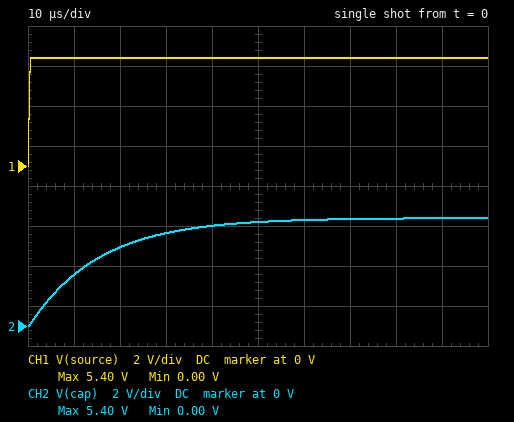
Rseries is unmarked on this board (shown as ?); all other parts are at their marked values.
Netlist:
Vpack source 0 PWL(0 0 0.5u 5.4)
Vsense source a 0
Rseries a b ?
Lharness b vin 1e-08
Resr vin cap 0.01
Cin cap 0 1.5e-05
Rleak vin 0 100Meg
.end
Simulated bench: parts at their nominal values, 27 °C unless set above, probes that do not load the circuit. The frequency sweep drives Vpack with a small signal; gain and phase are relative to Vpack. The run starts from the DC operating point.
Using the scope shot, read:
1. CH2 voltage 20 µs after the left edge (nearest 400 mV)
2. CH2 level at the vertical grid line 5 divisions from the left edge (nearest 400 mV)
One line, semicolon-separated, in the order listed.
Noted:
4.0 V; 5.2 V
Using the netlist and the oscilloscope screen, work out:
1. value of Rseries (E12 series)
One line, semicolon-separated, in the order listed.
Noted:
1 Ω
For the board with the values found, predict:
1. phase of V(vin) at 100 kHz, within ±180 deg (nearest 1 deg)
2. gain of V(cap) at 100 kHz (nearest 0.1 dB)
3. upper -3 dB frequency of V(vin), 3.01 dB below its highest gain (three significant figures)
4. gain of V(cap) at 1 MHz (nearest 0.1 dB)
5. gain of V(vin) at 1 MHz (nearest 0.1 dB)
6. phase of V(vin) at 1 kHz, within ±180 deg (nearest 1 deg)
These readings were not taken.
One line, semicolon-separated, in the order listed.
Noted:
-79 deg; -19.6 dB; 10.5 kHz; -39.6 dB; -36.8 dB; -5 deg
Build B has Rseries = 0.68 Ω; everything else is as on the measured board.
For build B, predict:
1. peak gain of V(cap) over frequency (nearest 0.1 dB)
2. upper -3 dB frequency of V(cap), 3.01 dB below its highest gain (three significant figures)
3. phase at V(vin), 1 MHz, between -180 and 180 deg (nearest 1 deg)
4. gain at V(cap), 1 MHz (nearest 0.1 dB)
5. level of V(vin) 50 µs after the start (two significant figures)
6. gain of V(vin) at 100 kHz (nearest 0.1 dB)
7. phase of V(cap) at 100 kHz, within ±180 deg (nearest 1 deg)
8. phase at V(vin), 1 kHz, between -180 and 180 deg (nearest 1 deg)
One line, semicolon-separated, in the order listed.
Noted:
0 dB; 15.4 kHz; -51 deg; -36.3 dB; 5.4 V; -16.3 dB; -82 deg; -4 deg
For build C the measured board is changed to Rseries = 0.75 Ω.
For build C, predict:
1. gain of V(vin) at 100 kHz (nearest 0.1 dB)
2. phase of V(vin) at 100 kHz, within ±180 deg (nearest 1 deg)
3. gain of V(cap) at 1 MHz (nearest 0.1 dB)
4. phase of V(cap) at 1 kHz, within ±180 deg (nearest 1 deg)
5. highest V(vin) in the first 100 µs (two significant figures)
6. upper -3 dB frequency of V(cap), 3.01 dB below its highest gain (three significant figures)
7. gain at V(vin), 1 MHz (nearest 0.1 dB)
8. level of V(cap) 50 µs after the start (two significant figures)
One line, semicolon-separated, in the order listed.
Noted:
-17.1 dB; -77 deg; -37.1 dB; -4 deg; 5.4 V; 14.0 kHz; -34.4 dB; 5.3 V
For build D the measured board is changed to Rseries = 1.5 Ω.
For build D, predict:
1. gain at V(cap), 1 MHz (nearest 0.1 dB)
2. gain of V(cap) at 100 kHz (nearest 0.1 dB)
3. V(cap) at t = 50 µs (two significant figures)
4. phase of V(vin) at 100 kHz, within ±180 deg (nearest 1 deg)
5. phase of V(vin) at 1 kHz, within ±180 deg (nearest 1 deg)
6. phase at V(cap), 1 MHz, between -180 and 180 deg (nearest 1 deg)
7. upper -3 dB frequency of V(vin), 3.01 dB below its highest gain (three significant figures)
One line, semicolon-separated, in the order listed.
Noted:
-43.1 dB; -23.1 dB; 4.8 V; -81 deg; -8 deg; -92 deg; 7.03 kHz
